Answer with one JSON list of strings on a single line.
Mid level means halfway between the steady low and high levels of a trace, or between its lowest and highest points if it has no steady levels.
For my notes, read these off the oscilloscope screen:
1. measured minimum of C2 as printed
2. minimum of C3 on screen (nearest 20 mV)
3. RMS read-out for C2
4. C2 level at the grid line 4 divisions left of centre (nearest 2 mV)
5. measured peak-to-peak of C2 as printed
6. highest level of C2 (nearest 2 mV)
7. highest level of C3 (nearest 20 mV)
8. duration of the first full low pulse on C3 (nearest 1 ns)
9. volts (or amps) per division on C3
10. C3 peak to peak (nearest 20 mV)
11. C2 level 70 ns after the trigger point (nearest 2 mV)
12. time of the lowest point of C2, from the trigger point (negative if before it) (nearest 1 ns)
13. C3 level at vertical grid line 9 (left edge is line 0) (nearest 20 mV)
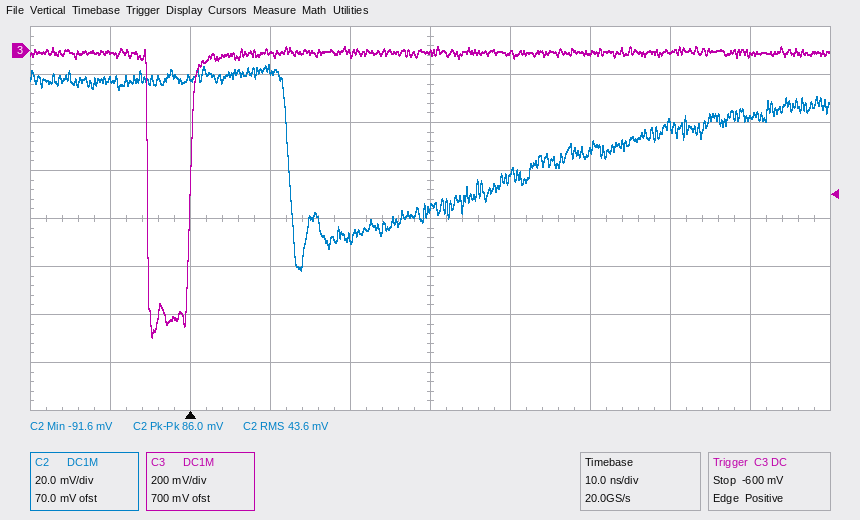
["-91.6 mV", "-1.20 V", "43.6 mV", "-12 mV", "86.0 mV", "-6 mV", "20 mV", "5 ns", "200 mV", "1.22 V", "-28 mV", "+14 ns", "-20 mV"]
